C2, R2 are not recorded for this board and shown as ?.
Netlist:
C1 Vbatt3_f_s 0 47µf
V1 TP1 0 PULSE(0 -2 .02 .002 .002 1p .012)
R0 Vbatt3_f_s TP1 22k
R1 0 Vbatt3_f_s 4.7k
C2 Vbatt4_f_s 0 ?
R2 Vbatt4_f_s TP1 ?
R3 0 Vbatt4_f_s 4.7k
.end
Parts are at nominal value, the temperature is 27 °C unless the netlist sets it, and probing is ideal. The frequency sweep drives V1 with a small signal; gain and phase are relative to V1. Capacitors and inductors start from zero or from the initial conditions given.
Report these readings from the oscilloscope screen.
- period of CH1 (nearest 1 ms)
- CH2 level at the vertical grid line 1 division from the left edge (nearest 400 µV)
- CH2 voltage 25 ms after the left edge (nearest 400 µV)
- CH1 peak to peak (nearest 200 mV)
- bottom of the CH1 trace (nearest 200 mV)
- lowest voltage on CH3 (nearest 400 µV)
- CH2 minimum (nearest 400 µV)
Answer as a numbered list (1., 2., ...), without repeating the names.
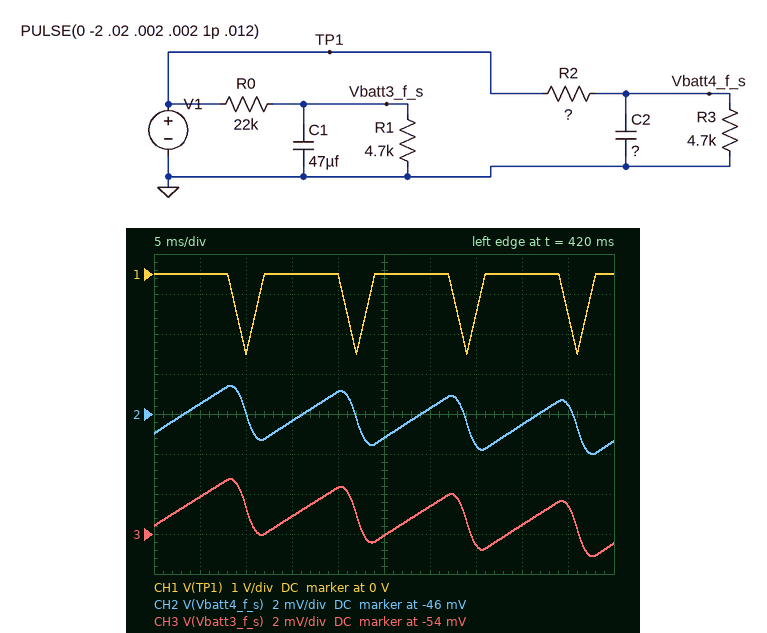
1. 12 ms
2. -45.6 mV
3. -47.2 mV
4. 2.0 V
5. -2.0 V
6. -55.2 mV
7. -48.0 mV
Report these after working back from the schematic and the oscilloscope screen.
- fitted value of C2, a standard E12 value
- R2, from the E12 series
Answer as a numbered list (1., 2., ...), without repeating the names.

1. 39 µF
2. 27 kΩ
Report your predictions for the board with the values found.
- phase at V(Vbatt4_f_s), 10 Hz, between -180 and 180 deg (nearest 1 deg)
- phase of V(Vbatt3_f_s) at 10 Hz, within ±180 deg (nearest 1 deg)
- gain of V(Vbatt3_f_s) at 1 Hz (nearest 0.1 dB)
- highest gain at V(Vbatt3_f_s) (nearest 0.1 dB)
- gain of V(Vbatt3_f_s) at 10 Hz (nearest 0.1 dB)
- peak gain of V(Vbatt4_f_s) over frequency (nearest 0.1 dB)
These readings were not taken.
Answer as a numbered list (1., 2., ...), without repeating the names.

1. -84 deg
2. -85 deg
3. -18.7 dB
4. -15.1 dB
5. -36.3 dB
6. -16.6 dB
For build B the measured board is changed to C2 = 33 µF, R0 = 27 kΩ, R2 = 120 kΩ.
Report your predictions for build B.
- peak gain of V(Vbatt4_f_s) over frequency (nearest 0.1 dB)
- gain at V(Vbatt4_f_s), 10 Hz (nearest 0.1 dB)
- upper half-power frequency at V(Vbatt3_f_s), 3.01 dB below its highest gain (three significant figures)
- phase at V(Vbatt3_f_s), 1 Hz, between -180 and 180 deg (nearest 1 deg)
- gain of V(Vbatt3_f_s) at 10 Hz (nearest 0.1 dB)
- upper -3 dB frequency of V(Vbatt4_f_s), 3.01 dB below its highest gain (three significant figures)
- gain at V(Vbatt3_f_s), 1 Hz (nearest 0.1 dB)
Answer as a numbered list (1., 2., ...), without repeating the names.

1. -28.5 dB
2. -48.0 dB
3. 846 mHz
4. -50 deg
5. -38.1 dB
6. 1.07 Hz
7. -20.4 dB
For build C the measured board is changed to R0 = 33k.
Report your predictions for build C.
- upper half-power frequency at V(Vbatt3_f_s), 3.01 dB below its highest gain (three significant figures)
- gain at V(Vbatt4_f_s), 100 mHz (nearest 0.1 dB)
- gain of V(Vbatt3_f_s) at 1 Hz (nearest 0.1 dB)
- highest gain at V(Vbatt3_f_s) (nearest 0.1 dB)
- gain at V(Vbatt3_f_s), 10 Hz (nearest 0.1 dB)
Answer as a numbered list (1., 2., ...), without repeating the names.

1. 823 mHz
2. -16.6 dB
3. -22.0 dB
4. -18.1 dB
5. -39.8 dB
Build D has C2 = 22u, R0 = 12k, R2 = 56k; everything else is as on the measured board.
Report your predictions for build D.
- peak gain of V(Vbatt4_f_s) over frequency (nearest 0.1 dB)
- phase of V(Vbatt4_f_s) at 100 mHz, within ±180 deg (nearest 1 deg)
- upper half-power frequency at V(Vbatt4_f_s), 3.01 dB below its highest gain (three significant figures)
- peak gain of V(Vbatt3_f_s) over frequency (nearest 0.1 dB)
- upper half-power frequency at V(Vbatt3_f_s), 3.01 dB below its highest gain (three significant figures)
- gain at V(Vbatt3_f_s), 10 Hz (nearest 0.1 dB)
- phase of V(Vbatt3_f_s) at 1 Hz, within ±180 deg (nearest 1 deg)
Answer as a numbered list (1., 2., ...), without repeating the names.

1. -22.2 dB
2. -3 deg
3. 1.67 Hz
4. -11.0 dB
5. 1.00 Hz
6. -31.0 dB
7. -45 deg
